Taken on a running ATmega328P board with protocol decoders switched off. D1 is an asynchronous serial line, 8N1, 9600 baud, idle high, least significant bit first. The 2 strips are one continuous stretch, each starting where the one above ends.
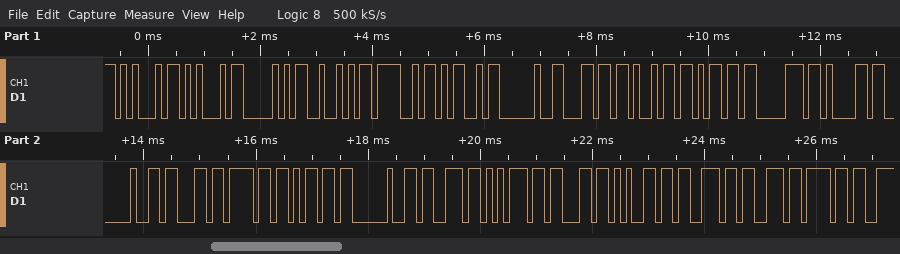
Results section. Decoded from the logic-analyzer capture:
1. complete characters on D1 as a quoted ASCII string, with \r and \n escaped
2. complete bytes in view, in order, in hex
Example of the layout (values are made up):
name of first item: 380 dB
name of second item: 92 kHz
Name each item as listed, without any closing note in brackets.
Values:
complete characters on D1 as a quoted ASCII string, with \r and \n escaped: "EEPROM limpa com sucesso"
complete bytes in view, in order, in hex: 45 45 50 52 4F 4D 20 6C 69 6D 70 61 20 63 6F 6D 20 73 75 63 65 73 73 6F
